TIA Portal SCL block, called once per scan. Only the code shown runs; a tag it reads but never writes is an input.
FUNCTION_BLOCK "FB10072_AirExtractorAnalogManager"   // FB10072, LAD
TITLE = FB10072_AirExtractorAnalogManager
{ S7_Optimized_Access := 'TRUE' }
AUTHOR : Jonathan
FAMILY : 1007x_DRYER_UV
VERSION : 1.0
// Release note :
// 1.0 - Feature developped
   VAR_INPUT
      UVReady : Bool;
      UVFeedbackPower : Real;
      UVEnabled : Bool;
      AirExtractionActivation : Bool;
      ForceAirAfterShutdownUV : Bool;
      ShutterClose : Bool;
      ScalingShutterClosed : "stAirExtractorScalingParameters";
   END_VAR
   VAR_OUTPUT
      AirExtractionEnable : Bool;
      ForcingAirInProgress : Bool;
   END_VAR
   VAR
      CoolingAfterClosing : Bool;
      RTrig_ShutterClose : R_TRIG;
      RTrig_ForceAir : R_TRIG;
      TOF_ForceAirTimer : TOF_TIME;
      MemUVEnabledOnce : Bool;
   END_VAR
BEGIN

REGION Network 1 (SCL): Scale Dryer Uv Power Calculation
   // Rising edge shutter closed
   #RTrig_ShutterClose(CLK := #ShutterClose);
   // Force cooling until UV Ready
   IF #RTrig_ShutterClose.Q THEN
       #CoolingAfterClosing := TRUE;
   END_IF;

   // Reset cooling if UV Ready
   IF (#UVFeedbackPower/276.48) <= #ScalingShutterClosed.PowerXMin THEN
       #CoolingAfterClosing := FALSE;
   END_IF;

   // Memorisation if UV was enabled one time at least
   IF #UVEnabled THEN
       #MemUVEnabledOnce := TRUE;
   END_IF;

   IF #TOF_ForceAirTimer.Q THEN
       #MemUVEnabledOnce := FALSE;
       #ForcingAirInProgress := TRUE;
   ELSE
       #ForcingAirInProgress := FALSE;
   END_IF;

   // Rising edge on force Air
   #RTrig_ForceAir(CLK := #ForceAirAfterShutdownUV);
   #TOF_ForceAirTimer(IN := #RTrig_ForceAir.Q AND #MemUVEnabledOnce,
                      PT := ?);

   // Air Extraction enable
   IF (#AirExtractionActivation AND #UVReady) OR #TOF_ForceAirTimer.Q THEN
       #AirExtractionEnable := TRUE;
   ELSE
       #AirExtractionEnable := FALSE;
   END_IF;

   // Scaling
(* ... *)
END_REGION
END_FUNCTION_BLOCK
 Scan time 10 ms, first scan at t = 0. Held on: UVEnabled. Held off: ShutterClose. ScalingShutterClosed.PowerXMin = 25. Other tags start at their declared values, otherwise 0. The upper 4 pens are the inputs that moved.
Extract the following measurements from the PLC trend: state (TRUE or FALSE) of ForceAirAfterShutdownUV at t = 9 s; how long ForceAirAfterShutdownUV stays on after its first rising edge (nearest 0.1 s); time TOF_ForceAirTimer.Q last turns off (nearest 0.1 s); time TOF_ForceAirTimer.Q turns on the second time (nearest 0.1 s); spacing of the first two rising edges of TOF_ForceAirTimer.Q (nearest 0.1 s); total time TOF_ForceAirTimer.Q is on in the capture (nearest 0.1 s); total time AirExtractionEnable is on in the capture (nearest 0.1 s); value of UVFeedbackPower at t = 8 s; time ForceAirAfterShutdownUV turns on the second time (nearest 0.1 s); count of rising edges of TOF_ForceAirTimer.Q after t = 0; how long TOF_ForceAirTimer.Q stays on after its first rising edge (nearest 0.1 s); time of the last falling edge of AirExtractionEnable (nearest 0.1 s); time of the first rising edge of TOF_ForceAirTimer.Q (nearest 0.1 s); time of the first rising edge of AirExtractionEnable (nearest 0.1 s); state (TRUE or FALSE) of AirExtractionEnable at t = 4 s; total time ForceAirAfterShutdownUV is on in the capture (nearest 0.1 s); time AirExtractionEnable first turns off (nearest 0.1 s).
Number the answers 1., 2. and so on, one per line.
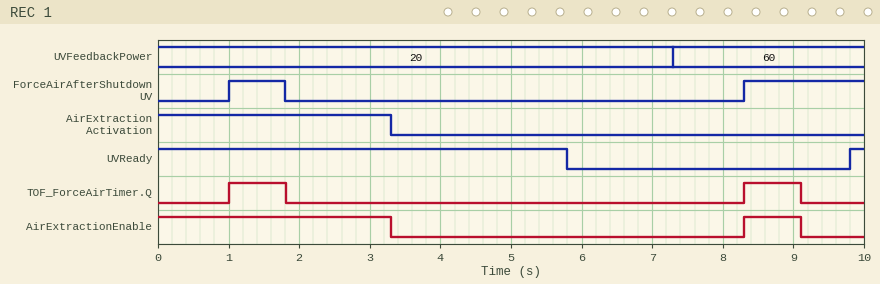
1. TRUE
2. 0.8 s
3. 9.1 s
4. 8.3 s
5. 7.3 s
6. 1.6 s
7. 4.1 s
8. 60
9. 8.3 s
10. 2
11. 0.8 s
12. 9.1 s
13. 1.0 s
14. 8.3 s
15. FALSE
16. 2.5 s
17. 3.3 s
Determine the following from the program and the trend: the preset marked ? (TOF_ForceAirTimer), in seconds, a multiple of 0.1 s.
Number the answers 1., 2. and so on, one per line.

1. 0.8 s
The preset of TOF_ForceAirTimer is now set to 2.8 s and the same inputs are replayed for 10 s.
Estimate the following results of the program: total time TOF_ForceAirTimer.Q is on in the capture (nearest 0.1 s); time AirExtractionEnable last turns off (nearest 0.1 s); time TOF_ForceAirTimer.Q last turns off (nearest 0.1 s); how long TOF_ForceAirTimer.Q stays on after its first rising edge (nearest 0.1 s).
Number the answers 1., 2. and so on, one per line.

1. 4.5 s
2. 3.8 s
3. 3.8 s
4. 2.8 s
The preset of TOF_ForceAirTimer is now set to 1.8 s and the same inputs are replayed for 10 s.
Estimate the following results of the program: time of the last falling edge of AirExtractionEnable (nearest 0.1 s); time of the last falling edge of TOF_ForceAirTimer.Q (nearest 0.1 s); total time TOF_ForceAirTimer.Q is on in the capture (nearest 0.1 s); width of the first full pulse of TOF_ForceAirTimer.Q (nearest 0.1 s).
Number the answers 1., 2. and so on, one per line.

1. 3.3 s
2. 2.8 s
3. 3.5 s
4. 1.8 s
